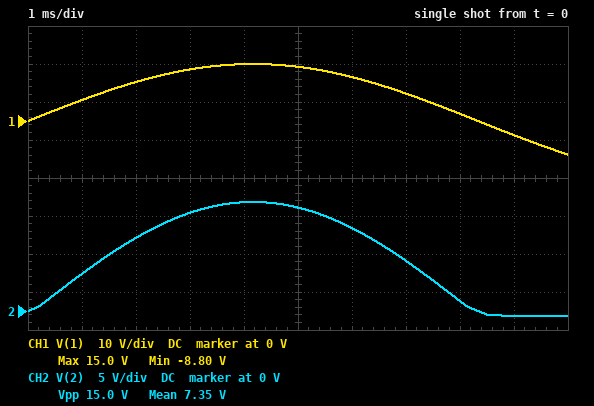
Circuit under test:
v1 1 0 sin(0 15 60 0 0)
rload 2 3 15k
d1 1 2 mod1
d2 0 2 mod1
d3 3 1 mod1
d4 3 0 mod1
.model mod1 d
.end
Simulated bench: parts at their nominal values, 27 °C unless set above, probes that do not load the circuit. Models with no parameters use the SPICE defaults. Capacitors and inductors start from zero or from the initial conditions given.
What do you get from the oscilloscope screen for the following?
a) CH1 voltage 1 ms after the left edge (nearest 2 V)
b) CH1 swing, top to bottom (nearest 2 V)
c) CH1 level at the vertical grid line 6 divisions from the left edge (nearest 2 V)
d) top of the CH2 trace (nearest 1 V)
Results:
6 V
24 V
12 V
14 V
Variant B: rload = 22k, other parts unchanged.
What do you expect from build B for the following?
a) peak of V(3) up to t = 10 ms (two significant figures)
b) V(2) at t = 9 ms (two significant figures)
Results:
640 mV
-600 mV
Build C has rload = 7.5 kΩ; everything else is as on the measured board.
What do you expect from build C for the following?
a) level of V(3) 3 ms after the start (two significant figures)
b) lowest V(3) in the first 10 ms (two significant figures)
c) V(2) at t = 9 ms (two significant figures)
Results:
670 mV
-8.2 V
-630 mV
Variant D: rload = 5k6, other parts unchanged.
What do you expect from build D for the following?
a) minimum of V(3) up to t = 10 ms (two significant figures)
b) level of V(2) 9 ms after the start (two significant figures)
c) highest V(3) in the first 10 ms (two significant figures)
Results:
-8.2 V
-630 mV
680 mV
